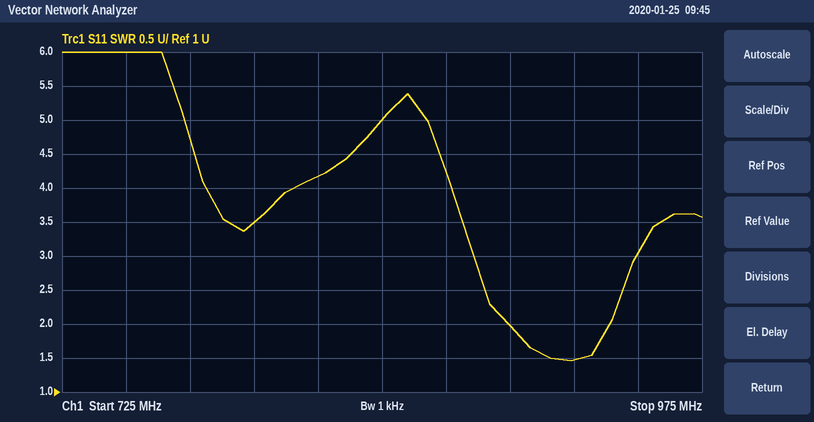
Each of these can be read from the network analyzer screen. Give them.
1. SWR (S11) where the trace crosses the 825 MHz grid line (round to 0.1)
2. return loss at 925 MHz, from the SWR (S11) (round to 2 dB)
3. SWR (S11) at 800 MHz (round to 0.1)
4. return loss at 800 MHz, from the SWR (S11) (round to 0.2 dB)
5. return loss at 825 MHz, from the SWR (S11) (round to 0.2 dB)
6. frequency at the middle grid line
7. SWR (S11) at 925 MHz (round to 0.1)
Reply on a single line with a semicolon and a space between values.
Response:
4.2; 14 dB; 3.5; 5.2 dB; 4.2 dB; 850 MHz; 1.5
